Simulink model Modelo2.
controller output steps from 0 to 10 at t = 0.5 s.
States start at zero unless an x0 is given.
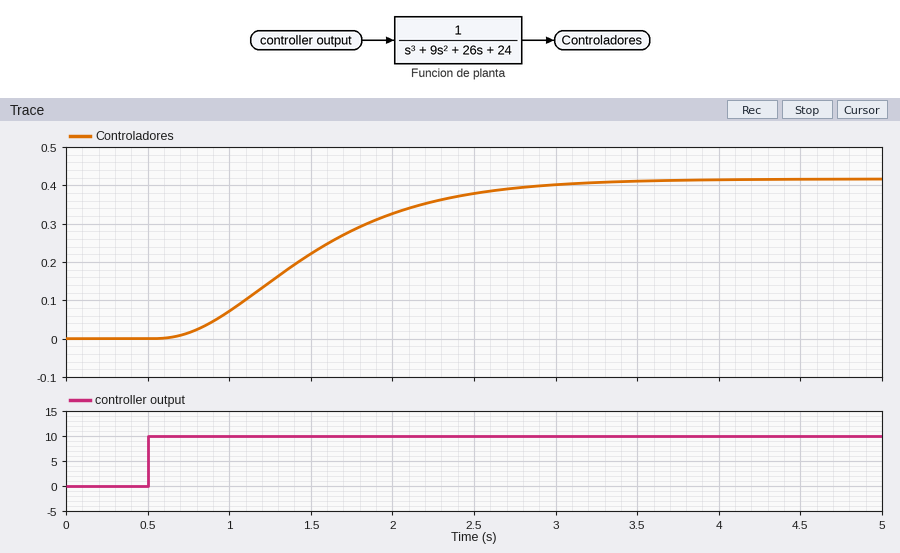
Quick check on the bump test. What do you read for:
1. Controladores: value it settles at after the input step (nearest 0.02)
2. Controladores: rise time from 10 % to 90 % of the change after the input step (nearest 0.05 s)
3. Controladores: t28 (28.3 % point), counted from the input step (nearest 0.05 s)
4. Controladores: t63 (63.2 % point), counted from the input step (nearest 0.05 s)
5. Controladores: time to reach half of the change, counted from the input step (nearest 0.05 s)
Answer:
0.42
1.55 s
0.65 s
1.15 s
0.95 s
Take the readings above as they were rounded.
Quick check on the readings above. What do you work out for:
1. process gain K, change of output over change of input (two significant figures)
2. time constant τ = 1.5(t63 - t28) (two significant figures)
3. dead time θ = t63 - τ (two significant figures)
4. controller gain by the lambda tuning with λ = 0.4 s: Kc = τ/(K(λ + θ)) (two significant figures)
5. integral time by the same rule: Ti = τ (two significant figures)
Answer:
0.042
0.75 s
0.40 s
22
0.75 s
